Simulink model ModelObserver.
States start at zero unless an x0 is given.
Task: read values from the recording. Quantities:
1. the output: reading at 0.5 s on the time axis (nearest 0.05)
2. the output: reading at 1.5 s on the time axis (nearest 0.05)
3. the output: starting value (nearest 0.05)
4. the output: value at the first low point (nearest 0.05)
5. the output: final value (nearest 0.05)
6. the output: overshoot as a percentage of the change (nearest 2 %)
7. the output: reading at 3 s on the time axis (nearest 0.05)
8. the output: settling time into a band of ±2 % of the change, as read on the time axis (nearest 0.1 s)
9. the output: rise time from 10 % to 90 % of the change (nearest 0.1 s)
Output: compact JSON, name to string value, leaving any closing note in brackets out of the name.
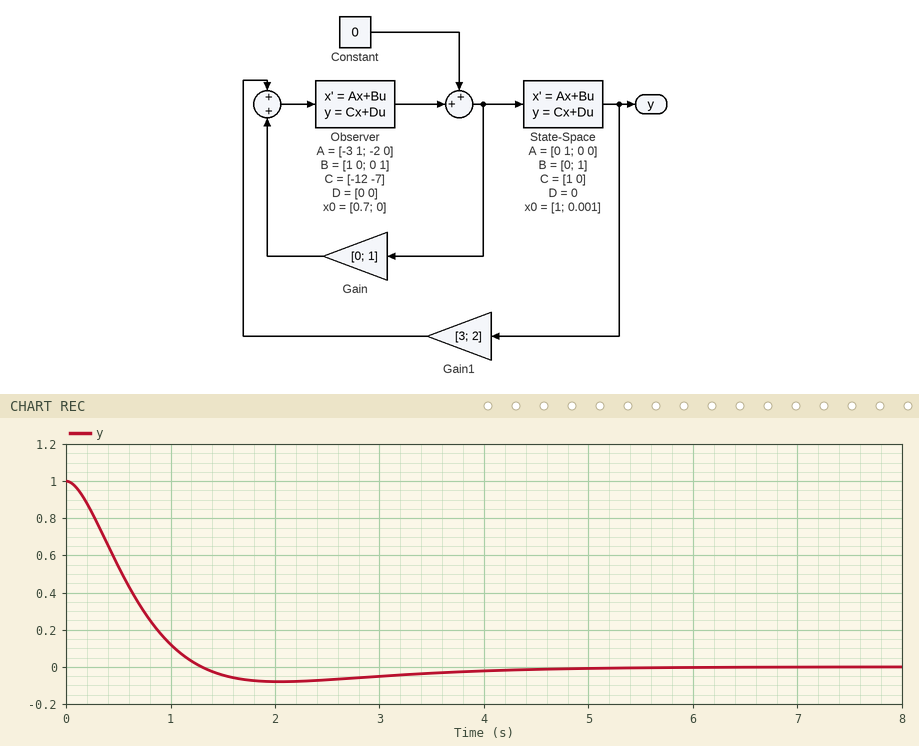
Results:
{"the output: reading at 0.5 s on the time axis": "0.55", "the output: reading at 1.5 s on the time axis": "-0.05", "the output: starting value": "1.00", "the output: value at the first low point": "-0.10", "the output: final value": "0.00", "the output: overshoot as a percentage of the change": "8 %", "the output: reading at 3 s on the time axis": "-0.05", "the output: settling time into a band of ±2 % of the change, as read on the time axis": "4.1 s", "the output: rise time from 10 % to 90 % of the change": "0.9 s"}
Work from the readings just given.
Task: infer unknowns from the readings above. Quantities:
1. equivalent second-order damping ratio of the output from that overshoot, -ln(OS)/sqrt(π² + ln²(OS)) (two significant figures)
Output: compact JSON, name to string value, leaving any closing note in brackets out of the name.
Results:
{"equivalent second-order damping ratio of the output from that overshoot, -ln(OS)/sqrt(π² + ln²(OS))": "0.63"}
